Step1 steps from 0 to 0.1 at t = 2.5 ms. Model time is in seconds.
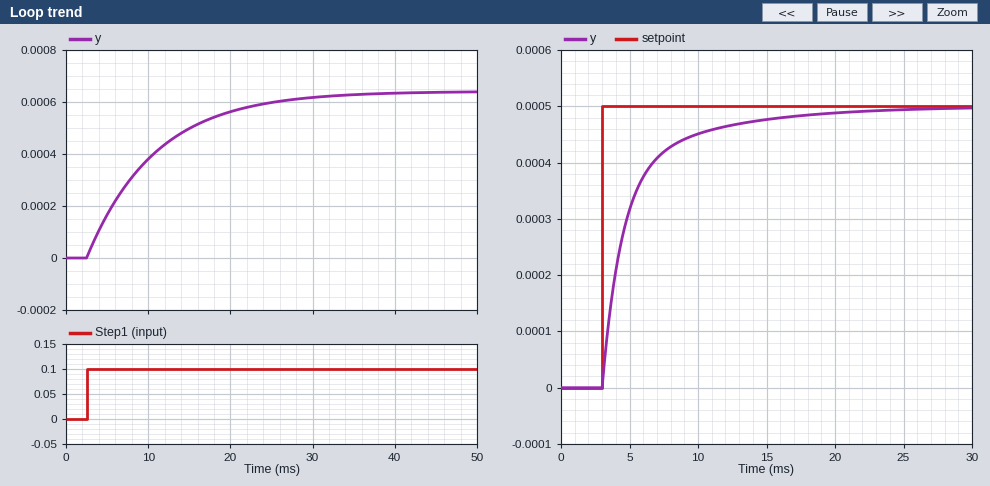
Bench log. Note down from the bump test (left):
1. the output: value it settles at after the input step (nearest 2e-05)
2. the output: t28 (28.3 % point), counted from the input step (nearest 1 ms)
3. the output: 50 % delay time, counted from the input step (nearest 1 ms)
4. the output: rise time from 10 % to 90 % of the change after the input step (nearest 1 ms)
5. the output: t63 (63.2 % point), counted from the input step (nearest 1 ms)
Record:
0.00064
3 ms
6 ms
18 ms
8 ms
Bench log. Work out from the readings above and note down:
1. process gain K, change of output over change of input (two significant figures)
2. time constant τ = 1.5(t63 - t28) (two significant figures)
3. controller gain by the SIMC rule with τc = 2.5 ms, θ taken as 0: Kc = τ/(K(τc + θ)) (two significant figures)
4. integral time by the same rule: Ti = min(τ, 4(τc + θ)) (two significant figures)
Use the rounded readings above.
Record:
0.0064
7.5 ms
470
7.5 ms
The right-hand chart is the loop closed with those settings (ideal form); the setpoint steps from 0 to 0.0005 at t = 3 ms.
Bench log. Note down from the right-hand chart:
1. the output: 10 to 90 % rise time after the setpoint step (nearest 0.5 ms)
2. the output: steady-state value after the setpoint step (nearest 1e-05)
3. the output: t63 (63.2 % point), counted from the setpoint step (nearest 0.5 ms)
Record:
6.5 ms
0.00050
2.0 ms
